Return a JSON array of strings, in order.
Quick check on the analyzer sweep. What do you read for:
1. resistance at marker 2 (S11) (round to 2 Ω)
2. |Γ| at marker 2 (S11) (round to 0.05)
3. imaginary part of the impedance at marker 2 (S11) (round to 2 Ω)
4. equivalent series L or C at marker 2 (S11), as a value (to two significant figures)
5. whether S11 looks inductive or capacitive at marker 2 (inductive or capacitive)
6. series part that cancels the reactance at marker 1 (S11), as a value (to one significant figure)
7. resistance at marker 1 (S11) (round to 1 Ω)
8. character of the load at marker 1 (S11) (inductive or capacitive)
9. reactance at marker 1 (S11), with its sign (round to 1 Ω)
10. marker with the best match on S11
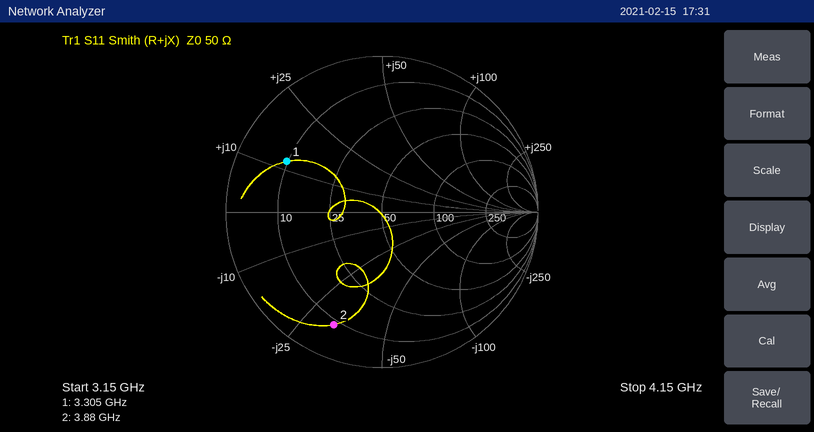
["8 Ω", "0.80", "-32 Ω", "1.3 pF", "capacitive", "4 pF", "10 Ω", "inductive", "+12 Ω", "marker 1"]
